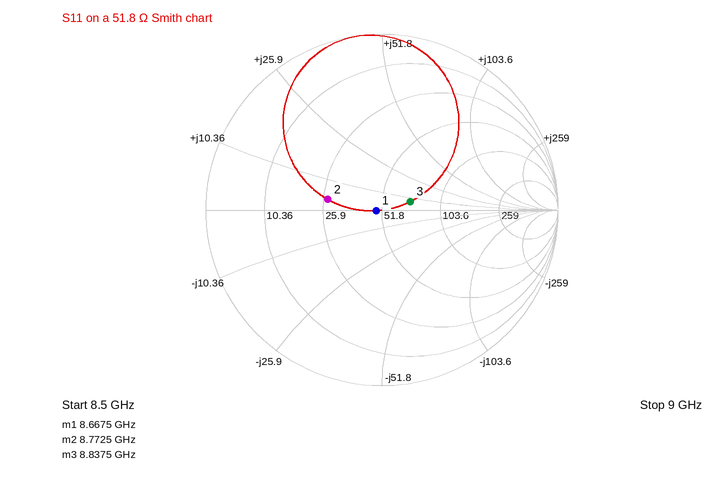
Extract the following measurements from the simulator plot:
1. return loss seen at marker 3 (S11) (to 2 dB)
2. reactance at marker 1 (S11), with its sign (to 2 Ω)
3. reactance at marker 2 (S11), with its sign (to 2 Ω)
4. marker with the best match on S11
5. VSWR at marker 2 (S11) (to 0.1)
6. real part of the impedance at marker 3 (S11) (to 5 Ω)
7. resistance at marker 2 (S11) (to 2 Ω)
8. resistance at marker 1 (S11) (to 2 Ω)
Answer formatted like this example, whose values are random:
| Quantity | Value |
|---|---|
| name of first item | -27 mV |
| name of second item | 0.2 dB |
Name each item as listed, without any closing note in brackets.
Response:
| Quantity | Value |
|---|---|
| return loss seen at marker 3 (S11) | 16 dB |
| reactance at marker 1 (S11), with its sign | 0 Ω |
| reactance at marker 2 (S11), with its sign | +4 Ω |
| marker with the best match on S11 | marker 1 |
| VSWR at marker 2 (S11) | 1.9 |
| real part of the impedance at marker 3 (S11) | 70 Ω |
| resistance at marker 2 (S11) | 28 Ω |
| resistance at marker 1 (S11) | 48 Ω |
